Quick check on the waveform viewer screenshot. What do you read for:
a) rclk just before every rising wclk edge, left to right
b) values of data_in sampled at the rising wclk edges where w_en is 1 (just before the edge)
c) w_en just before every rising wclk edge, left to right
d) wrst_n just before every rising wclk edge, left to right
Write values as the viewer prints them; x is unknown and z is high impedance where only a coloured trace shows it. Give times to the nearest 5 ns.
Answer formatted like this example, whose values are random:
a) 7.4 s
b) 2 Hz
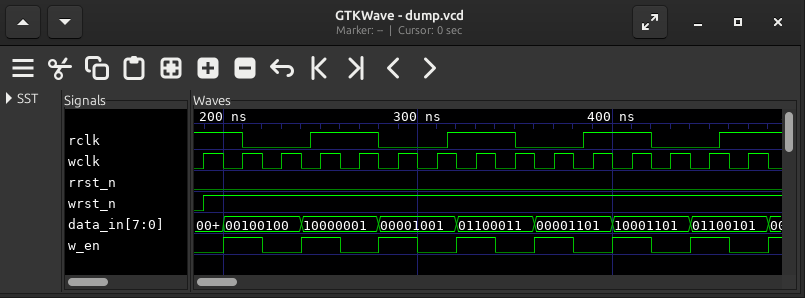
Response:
a) 1 1 0 1 1 0 0 1 1 0 1 1 0 0 1
b) 00100100, 10000001, 00001001, 01100011, 00001101, 10001101, 01100101
c) 0 1 0 1 0 1 0 1 0 1 0 1 0 1 0
d) 0 1 1 1 1 1 1 1 1 1 1 1 1 1 1
